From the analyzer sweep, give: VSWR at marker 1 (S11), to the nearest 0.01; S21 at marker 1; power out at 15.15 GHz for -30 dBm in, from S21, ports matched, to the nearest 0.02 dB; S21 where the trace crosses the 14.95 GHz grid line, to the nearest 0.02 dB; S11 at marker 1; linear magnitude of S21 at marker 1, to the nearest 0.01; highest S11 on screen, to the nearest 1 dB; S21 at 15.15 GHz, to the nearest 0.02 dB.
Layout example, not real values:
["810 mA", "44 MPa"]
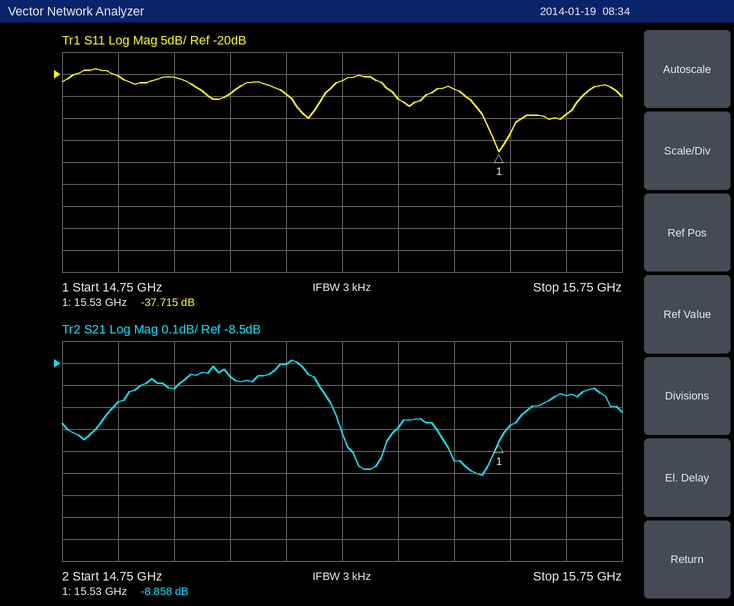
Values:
["1.03", "-8.858 dB", "-38.50 dBm", "-8.62 dB", "-37.715 dB", "0.36", "-19 dB", "-8.50 dB"]
